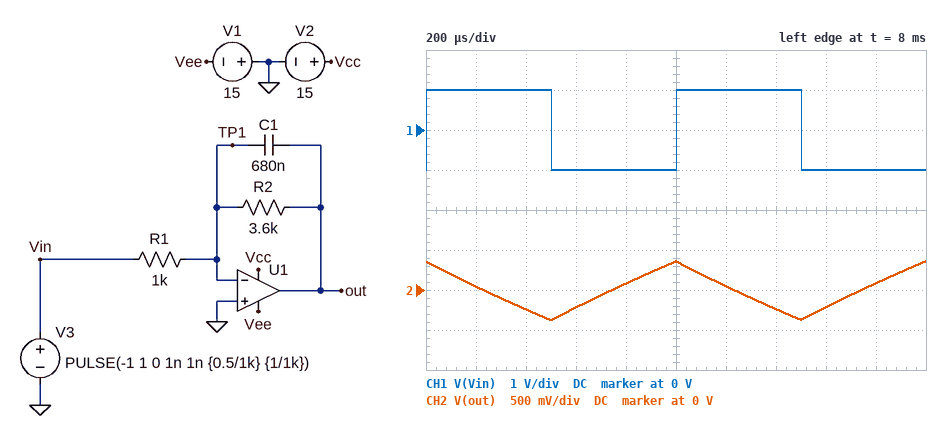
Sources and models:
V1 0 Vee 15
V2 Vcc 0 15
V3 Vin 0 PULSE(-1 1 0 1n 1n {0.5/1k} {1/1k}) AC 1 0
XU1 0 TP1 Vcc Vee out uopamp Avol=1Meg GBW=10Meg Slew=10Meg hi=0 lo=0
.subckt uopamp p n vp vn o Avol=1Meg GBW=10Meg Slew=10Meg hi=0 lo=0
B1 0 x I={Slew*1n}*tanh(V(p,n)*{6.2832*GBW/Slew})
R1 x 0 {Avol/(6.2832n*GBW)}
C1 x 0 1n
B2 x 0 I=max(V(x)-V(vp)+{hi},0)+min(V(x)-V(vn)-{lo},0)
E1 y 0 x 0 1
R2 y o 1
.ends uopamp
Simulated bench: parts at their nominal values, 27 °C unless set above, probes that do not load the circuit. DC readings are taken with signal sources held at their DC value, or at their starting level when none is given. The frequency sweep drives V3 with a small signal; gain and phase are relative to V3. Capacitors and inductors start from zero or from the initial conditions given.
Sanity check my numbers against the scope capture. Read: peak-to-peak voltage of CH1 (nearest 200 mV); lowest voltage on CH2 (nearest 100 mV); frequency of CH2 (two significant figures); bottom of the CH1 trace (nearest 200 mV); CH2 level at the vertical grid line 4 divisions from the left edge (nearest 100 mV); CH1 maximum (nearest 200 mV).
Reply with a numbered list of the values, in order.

1. 2.0 V
2. -400 mV
3. 1.0 kHz
4. -1.0 V
5. 100 mV
6. 1.0 V
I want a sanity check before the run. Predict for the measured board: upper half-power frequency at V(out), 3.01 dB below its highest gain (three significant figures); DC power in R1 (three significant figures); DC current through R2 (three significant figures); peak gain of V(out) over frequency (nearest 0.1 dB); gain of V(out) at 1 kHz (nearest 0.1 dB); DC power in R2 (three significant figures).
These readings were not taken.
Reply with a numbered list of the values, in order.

1. 65.0 Hz
2. 1.00 mW
3. 1.00 mA
4. 11.1 dB
5. -12.6 dB
6. 3.60 mW
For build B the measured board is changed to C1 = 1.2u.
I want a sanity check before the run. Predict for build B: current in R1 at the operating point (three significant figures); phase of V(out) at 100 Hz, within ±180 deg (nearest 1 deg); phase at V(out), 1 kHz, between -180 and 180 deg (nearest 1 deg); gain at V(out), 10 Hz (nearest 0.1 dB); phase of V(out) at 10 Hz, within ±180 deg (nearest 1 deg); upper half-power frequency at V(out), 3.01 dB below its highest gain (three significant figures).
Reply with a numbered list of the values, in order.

1. 1.00 mA
2. 110 deg
3. 92 deg
4. 10.8 dB
5. 165 deg
6. 36.8 Hz
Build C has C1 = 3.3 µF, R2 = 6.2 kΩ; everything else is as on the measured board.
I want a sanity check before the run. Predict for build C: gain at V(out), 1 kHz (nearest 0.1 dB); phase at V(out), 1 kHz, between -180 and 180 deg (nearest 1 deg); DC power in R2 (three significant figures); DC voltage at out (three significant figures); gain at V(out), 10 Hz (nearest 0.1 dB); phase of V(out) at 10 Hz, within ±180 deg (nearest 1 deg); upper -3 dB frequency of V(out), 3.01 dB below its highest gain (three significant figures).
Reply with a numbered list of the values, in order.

1. -26.3 dB
2. 90 deg
3. 6.20 mW
4. 6.20 V
5. 11.6 dB
6. 128 deg
7. 7.78 Hz
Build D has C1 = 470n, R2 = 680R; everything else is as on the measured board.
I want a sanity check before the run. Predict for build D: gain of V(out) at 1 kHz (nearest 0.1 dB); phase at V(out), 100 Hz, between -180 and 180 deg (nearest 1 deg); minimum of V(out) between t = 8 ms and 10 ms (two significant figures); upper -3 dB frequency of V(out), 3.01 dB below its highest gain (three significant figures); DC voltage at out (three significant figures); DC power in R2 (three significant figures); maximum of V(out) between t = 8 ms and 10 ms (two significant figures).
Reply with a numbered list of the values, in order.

1. -10.4 dB
2. 169 deg
3. -450 mV
4. 498 Hz
5. 680 mV
6. 680 µW
7. 450 mV
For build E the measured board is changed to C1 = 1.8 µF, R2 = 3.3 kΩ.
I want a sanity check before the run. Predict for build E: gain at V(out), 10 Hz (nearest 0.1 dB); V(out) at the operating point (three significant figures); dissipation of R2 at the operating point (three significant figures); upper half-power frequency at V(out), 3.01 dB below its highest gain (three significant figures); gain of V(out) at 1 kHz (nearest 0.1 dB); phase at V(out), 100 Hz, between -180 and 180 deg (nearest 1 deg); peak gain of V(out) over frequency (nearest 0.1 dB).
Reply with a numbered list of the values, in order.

1. 9.8 dB
2. 3.30 V
3. 3.30 mW
4. 26.8 Hz
5. -21.1 dB
6. 105 deg
7. 10.4 dB
